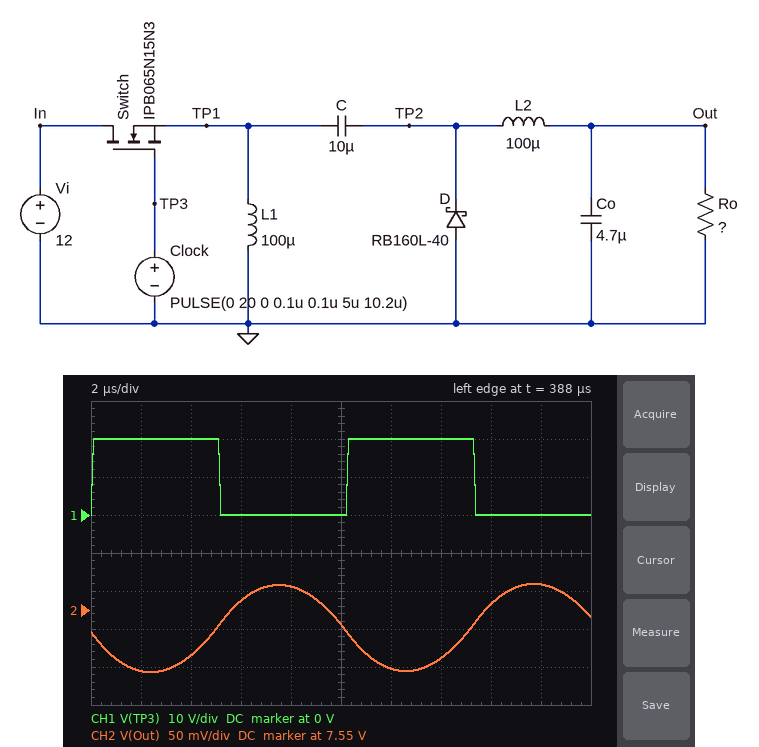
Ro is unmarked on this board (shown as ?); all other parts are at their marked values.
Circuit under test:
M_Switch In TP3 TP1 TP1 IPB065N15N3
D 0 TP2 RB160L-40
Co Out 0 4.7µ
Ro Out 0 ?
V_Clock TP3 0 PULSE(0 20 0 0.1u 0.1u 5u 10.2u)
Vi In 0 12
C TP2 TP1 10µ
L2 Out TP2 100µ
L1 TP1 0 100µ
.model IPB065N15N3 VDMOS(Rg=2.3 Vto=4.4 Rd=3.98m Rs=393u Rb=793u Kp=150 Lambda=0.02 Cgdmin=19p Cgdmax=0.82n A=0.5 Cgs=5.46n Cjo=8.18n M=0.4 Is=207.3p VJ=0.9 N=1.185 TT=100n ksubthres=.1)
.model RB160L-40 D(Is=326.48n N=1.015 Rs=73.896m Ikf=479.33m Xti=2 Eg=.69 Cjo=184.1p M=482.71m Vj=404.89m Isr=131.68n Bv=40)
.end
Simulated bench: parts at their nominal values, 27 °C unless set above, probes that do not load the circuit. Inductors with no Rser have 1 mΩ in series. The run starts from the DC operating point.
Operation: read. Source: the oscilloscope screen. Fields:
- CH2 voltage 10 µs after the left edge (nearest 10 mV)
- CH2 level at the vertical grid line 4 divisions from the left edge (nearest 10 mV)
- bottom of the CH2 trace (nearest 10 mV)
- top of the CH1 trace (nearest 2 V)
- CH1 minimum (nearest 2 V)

7.53 V
7.58 V
7.47 V
20 V
0 V
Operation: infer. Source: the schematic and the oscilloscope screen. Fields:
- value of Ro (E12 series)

4.7 Ω
